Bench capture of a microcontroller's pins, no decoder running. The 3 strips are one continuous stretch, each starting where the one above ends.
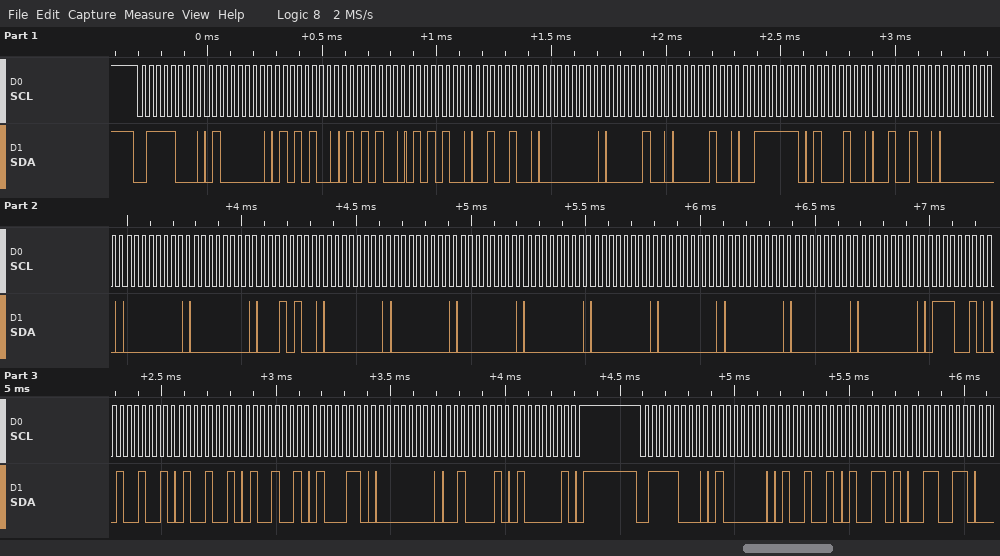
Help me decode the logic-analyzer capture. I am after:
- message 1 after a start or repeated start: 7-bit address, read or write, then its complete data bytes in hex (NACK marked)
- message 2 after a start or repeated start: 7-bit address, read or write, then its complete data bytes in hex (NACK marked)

0x3C write: 40 54 54 54 24 00 04 04 3F 44 24 00 00 00 14 00 00 00 00 00 00 00 00 00 72 49 49 49 46 00 21 41
0x3C write: 40 49 4D 33
